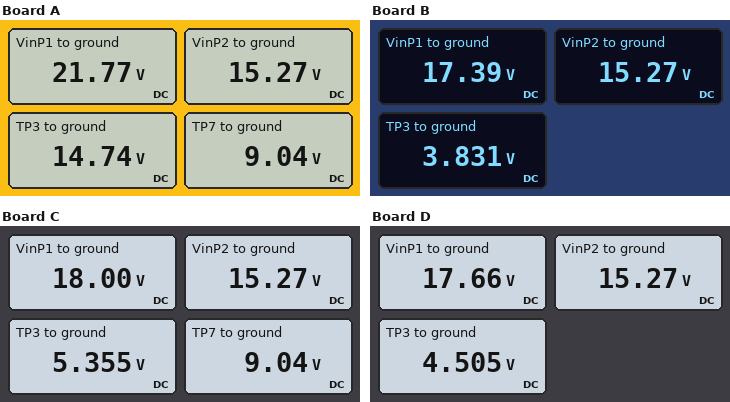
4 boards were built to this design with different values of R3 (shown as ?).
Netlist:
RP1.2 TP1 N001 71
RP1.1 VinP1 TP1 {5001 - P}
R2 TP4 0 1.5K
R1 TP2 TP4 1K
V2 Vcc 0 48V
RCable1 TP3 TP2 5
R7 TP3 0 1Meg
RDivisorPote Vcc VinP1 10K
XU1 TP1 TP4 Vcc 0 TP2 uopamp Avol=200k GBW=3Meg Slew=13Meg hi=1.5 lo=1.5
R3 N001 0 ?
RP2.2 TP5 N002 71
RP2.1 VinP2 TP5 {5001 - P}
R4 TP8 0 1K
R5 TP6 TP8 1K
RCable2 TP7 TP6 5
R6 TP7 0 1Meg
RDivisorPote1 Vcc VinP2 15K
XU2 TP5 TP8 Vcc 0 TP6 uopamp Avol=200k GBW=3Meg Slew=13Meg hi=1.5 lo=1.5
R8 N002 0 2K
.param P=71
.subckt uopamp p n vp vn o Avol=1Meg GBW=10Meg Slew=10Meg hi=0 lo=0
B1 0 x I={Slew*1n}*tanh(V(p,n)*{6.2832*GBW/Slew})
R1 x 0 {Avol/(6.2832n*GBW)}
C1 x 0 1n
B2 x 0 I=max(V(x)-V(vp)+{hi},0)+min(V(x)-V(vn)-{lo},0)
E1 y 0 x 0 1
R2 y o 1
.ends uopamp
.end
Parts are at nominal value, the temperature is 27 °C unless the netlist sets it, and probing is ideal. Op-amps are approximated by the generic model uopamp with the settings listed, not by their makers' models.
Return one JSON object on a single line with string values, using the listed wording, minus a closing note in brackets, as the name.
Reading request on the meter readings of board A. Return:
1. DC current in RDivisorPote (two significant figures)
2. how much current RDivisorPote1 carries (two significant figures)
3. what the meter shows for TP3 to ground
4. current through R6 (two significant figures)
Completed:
{"DC current in RDivisorPote": "2.6 mA", "how much current RDivisorPote1 carries": "2.2 mA", "what the meter shows for TP3 to ground": "14.74 V", "current through R6": "9.0 µA"}
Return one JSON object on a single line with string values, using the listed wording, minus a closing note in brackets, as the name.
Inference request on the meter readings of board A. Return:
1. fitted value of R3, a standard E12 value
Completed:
{"fitted value of R3, a standard E12 value": "3.3 kΩ"}
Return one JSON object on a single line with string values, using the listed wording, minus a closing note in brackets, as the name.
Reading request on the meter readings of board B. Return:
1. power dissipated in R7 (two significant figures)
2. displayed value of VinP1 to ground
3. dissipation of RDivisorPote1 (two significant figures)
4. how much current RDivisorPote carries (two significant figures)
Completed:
{"power dissipated in R7": "15 µW", "displayed value of VinP1 to ground": "17.39 V", "dissipation of RDivisorPote1": "71 mW", "how much current RDivisorPote carries": "3.1 mA"}
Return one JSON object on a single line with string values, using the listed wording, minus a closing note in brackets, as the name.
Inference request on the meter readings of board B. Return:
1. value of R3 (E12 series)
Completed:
{"value of R3": "680 Ω"}
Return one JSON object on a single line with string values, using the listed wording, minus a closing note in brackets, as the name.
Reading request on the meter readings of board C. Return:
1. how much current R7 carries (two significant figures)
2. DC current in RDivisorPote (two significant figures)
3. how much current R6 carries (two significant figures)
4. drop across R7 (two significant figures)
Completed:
{"how much current R7 carries": "5.4 µA", "DC current in RDivisorPote": "3.0 mA", "how much current R6 carries": "9.0 µA", "drop across R7": "5.4 V"}
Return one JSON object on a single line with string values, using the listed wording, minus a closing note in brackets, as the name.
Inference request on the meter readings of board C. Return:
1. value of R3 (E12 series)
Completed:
{"value of R3": "1 kΩ"}
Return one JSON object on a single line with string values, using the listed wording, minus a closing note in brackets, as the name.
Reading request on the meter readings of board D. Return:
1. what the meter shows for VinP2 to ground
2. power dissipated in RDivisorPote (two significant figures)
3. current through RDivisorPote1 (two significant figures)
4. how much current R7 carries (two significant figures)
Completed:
{"what the meter shows for VinP2 to ground": "15.27 V", "power dissipated in RDivisorPote": "92 mW", "current through RDivisorPote1": "2.2 mA", "how much current R7 carries": "4.5 µA"}
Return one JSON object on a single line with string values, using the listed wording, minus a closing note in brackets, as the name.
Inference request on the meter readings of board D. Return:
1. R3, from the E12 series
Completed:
{"R3, from the E12 series": "820 Ω"}
